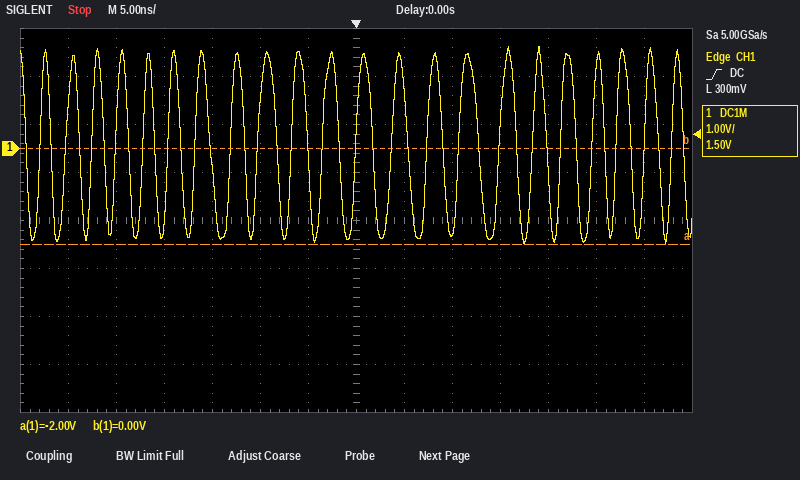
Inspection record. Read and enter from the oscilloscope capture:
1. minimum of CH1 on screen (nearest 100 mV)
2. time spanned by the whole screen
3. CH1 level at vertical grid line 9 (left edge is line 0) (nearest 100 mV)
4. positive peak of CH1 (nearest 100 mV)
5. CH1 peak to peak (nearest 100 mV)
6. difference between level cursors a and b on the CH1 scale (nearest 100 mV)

-2.0 V
70 ns
-1.7 V
2.1 V
4.1 V
2.0 V
